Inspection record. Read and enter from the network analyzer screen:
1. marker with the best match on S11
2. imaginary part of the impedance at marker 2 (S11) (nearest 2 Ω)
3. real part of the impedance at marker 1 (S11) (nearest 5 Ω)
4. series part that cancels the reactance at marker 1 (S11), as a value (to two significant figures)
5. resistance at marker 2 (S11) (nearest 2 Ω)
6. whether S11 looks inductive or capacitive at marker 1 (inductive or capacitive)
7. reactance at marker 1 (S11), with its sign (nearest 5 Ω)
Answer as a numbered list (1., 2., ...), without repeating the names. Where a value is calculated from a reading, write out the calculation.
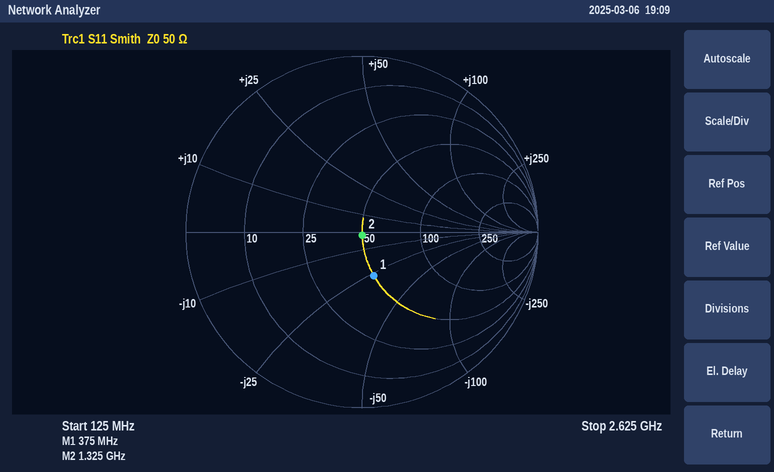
1. marker 2
2. -2 Ω
3. 50 Ω
4. L = 25 Ω/(2π × 375 MHz) ≈ 11 nH
5. 50 Ω
6. capacitive
7. -25 Ω
